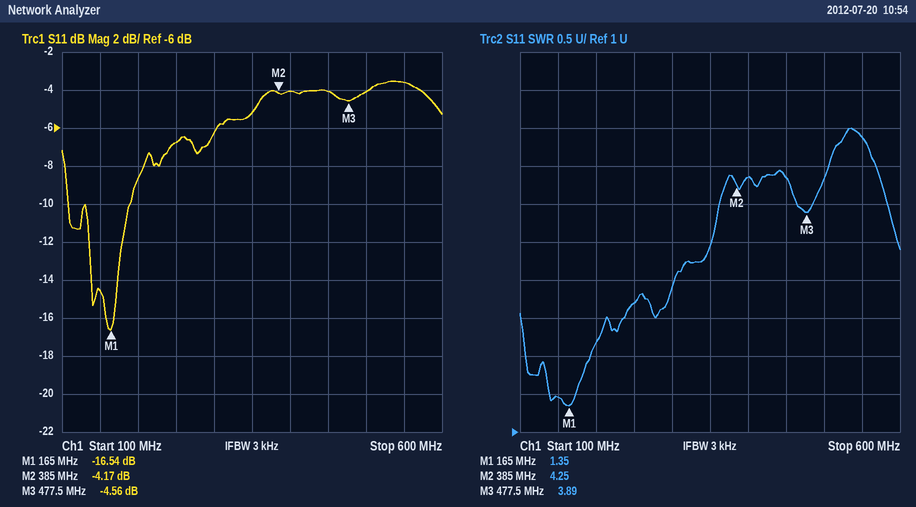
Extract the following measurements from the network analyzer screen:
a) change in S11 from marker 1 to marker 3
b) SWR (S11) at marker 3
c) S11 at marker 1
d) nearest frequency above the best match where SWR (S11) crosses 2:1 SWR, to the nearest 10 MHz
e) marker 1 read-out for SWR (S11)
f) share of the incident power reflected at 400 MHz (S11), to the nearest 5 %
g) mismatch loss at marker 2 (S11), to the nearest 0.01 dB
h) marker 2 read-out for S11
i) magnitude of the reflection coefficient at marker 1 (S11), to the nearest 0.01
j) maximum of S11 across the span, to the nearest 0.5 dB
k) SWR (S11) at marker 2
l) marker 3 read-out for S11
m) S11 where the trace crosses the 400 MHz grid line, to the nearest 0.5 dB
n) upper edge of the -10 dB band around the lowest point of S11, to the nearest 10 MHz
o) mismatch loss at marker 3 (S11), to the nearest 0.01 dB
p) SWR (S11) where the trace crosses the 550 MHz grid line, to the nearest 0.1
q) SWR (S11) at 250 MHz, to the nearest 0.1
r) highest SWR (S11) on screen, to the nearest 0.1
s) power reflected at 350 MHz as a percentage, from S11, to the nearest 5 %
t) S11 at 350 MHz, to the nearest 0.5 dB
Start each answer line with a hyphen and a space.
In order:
- 11.98 dB
- 3.89
- -16.54 dB
- 190 MHz
- 1.35
- 40 %
- 2.10 dB
- -4.17 dB
- 0.15
- -3.5 dB
- 4.25
- -4.56 dB
- -4.0 dB
- 190 MHz
- 1.87 dB
- 4.9
- 2.7
- 5.0
- 30 %
- -5.0 dB
